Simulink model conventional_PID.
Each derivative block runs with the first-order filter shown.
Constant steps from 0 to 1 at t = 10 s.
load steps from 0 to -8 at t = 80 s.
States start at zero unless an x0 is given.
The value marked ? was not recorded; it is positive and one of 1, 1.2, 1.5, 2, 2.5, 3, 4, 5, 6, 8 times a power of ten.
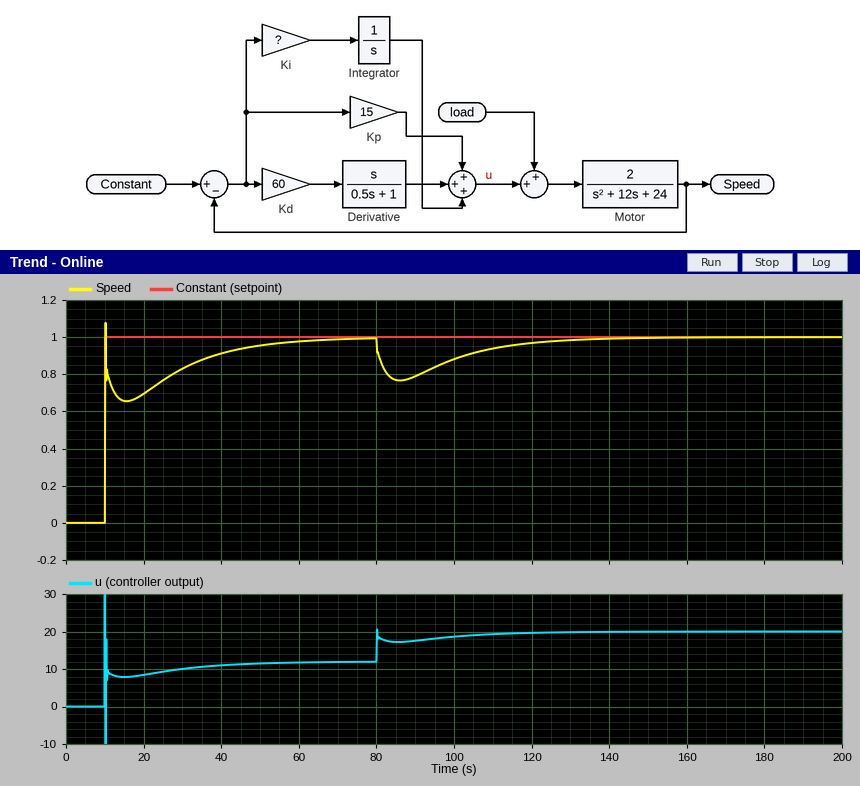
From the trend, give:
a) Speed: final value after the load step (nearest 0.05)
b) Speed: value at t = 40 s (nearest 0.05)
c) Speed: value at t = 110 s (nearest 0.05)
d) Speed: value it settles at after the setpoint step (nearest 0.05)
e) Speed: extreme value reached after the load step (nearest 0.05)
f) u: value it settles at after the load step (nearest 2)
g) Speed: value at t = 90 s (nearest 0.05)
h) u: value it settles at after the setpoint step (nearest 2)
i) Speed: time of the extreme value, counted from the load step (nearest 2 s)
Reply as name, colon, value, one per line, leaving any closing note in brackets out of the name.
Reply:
Speed: final value after the load step: 1.00
Speed: value at t = 40 s: 0.90
Speed: value at t = 110 s: 0.95
Speed: value it settles at after the setpoint step: 1.00
Speed: extreme value reached after the load step: 0.75
u: value it settles at after the load step: 20
Speed: value at t = 90 s: 0.80
u: value it settles at after the setpoint step: 12
Speed: time of the extreme value, counted from the load step: 6 s
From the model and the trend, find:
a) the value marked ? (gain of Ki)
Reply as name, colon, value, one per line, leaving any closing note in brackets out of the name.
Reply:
the value marked ?: 1.5
